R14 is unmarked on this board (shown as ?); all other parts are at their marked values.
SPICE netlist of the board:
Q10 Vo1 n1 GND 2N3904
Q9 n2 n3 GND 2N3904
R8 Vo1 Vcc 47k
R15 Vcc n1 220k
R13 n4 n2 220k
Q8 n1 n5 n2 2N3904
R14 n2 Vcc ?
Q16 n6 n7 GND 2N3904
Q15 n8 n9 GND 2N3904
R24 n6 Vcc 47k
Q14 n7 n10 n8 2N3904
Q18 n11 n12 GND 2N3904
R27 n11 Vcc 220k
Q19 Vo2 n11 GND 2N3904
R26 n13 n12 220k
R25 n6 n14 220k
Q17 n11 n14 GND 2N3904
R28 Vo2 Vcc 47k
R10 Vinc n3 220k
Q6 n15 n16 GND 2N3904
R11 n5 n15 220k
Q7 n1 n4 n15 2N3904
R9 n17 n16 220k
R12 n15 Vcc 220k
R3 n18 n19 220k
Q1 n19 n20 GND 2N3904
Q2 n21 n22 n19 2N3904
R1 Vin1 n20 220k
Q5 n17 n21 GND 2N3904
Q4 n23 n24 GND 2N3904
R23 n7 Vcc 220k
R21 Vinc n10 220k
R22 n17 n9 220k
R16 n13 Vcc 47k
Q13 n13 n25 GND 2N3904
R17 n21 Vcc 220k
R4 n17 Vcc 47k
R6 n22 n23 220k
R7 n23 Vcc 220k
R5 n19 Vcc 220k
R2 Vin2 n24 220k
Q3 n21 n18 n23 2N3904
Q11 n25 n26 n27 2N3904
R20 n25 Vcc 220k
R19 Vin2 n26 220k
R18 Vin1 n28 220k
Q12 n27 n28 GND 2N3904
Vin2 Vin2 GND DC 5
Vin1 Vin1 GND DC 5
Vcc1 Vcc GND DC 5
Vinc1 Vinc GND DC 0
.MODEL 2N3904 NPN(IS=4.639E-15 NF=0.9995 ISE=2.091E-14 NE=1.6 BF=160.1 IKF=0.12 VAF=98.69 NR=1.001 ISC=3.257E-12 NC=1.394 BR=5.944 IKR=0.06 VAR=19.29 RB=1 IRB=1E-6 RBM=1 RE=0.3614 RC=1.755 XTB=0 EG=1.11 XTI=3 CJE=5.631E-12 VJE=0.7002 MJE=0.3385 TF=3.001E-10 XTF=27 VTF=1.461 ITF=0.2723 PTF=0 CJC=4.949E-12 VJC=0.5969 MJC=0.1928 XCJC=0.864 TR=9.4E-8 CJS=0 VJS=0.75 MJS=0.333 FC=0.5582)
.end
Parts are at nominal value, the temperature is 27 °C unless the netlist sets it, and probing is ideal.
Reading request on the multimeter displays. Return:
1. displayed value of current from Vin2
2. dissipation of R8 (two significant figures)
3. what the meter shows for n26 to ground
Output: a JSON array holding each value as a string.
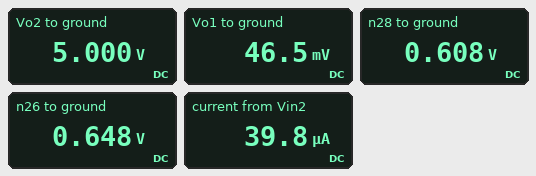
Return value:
["39.8 µA", "520 µW", "0.648 V"]
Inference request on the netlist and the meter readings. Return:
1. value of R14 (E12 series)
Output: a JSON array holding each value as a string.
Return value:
["180 kΩ"]
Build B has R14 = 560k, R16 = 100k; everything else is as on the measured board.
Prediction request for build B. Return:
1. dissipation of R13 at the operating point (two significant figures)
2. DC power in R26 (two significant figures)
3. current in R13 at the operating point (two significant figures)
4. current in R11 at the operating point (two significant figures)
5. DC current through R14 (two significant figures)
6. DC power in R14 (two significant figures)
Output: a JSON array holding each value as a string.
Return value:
["1.3 µW", "42 µW", "2.4 µA", "8.4 µA", "6.0 µA", "20 µW"]
